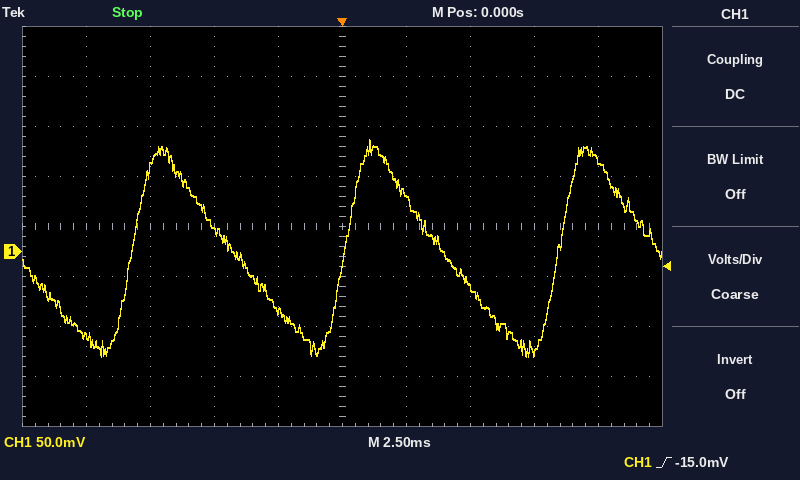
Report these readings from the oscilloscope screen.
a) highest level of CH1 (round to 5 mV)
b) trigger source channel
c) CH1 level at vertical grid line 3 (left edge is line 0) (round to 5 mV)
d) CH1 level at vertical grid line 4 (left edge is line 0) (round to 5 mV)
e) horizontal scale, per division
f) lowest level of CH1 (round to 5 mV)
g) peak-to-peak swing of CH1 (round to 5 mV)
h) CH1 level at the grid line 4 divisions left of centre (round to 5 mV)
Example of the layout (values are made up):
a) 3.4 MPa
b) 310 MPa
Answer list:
a) 110 mV
b) CH1
c) 20 mV
d) -60 mV
e) 2.5 ms
f) -105 mV
g) 215 mV
h) -85 mV
